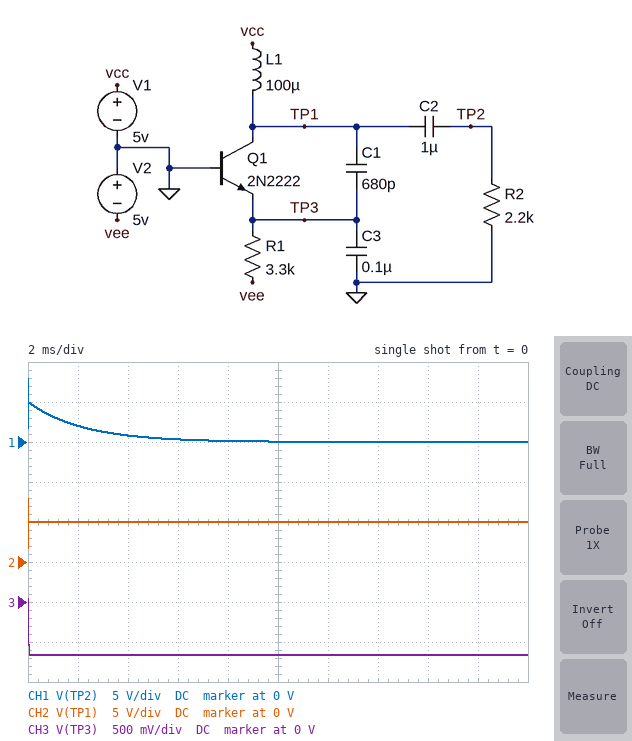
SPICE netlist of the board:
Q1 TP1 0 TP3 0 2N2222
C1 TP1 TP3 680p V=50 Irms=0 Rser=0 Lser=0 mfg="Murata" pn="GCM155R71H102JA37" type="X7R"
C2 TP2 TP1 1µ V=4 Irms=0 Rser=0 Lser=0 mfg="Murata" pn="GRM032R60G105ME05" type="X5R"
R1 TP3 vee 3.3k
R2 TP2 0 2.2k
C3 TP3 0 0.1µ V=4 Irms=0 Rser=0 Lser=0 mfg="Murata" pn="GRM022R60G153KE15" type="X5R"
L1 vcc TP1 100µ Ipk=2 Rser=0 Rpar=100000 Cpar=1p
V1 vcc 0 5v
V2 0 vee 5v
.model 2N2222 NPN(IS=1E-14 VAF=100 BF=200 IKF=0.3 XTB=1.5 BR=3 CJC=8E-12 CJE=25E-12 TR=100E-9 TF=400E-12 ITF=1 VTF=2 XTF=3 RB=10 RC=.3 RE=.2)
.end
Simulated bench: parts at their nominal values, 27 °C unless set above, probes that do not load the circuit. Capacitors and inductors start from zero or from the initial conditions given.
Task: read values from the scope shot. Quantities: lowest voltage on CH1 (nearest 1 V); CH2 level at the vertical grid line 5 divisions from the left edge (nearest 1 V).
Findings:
0 V
5 V
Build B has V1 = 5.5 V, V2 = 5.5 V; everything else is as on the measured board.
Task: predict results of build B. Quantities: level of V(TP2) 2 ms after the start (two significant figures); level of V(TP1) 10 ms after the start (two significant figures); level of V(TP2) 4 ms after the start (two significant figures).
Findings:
2.2 V
5.5 V
890 mV
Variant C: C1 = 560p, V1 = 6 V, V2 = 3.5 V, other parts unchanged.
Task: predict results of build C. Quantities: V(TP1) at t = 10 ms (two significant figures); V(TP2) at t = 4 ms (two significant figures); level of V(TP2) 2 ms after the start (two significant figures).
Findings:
6.0 V
970 mV
2.4 V
